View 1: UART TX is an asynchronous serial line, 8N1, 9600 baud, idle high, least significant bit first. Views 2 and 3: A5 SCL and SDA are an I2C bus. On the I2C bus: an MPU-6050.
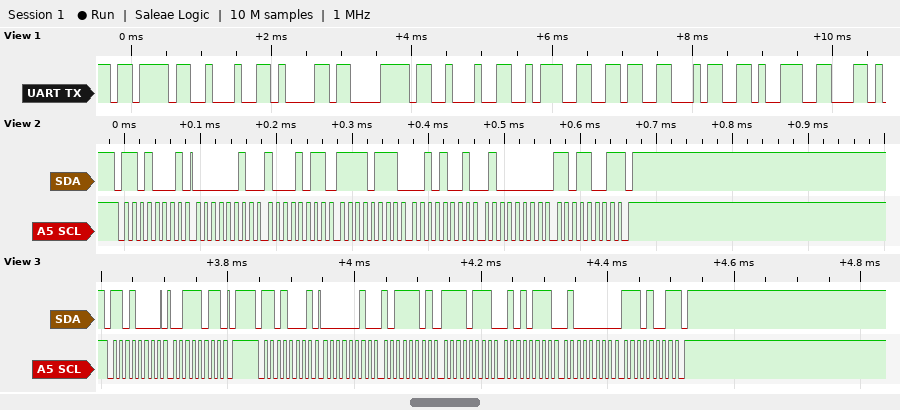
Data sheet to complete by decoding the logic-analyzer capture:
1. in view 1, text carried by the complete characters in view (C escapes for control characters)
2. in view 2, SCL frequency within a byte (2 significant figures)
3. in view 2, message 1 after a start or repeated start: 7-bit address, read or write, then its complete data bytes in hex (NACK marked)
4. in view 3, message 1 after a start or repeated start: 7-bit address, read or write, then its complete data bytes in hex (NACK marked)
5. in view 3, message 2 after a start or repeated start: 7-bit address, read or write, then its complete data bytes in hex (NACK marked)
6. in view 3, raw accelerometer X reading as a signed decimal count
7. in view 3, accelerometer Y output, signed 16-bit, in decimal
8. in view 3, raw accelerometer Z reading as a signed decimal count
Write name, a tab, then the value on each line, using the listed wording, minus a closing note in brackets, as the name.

in view 1, text carried by the complete characters in view	"{\"ax\":649"
in view 2, SCL frequency within a byte	100 kHz
in view 2, message 1 after a start or repeated start: 7-bit address, read or write, then its complete data bytes in hex	0x68 read: 02 8B F7 29 40 D9 NACK
in view 3, message 1 after a start or repeated start: 7-bit address, read or write, then its complete data bytes in hex	0x68 write: 3B
in view 3, message 2 after a start or repeated start: 7-bit address, read or write, then its complete data bytes in hex	0x68 read: 02 BD F7 57 40 E9 NACK
in view 3, raw accelerometer X reading as a signed decimal count	701
in view 3, accelerometer Y output, signed 16-bit, in decimal	-2217
in view 3, raw accelerometer Z reading as a signed decimal count	16617
